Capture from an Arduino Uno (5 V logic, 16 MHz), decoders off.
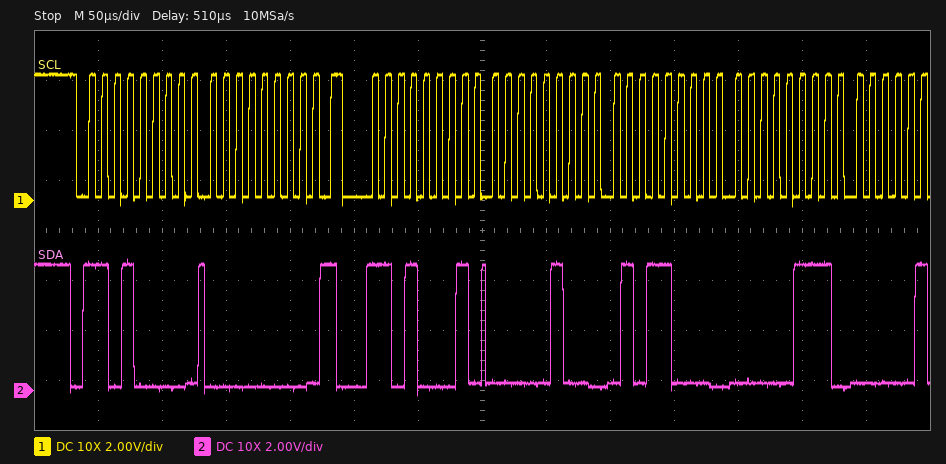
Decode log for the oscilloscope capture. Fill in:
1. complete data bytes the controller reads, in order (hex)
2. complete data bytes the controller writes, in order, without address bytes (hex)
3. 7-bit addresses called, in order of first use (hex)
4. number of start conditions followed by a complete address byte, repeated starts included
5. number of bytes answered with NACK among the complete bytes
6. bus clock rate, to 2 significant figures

04 58 07
00
0x68
2
0
100 kHz
